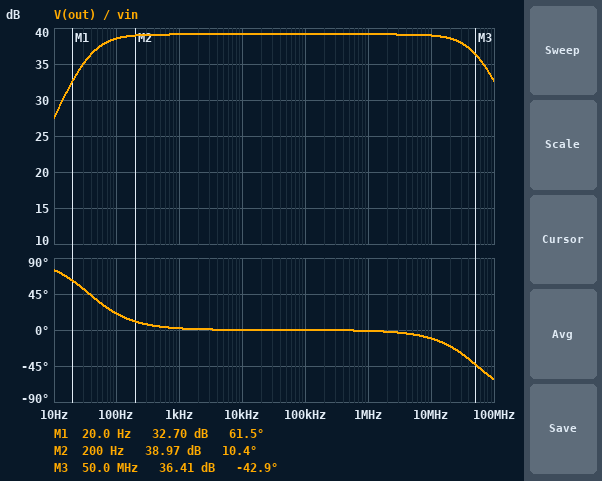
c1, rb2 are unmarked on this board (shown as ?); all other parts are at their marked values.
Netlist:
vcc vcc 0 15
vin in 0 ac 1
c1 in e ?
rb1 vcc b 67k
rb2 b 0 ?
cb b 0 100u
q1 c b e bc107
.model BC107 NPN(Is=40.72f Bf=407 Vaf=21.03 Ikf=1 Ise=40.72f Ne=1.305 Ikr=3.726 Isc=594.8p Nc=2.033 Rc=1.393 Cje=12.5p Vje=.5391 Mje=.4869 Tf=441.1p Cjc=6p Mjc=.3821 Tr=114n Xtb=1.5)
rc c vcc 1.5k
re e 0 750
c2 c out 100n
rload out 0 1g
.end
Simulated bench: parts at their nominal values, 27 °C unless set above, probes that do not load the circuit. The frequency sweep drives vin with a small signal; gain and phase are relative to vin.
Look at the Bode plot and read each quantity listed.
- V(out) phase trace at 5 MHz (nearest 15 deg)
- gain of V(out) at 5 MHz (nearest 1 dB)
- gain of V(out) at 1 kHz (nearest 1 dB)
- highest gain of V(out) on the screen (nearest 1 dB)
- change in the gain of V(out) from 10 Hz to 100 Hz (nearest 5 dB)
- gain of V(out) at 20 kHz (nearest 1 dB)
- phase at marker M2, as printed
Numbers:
0 deg
39 dB
39 dB
39 dB
10 dB
39 dB
10.4 deg
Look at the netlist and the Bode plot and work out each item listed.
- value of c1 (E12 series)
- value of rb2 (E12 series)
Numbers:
270 µF
10 kΩ
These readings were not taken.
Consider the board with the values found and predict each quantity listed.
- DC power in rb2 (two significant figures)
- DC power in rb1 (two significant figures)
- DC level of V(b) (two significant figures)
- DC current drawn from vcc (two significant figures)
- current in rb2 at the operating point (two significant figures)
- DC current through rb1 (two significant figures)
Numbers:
360 µW
2.6 mW
1.9 V
1.9 mA
190 µA
200 µA
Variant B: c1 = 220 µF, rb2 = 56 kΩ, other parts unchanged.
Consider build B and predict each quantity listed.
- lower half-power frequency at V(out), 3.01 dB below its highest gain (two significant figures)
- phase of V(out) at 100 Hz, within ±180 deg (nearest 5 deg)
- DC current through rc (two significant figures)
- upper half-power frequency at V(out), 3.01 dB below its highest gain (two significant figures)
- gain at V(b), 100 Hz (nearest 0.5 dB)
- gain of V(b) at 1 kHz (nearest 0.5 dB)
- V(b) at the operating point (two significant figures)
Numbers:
180 Hz
60 deg
6.6 mA
9.8 MHz
-11.0 dB
-24.5 dB
5.6 V
